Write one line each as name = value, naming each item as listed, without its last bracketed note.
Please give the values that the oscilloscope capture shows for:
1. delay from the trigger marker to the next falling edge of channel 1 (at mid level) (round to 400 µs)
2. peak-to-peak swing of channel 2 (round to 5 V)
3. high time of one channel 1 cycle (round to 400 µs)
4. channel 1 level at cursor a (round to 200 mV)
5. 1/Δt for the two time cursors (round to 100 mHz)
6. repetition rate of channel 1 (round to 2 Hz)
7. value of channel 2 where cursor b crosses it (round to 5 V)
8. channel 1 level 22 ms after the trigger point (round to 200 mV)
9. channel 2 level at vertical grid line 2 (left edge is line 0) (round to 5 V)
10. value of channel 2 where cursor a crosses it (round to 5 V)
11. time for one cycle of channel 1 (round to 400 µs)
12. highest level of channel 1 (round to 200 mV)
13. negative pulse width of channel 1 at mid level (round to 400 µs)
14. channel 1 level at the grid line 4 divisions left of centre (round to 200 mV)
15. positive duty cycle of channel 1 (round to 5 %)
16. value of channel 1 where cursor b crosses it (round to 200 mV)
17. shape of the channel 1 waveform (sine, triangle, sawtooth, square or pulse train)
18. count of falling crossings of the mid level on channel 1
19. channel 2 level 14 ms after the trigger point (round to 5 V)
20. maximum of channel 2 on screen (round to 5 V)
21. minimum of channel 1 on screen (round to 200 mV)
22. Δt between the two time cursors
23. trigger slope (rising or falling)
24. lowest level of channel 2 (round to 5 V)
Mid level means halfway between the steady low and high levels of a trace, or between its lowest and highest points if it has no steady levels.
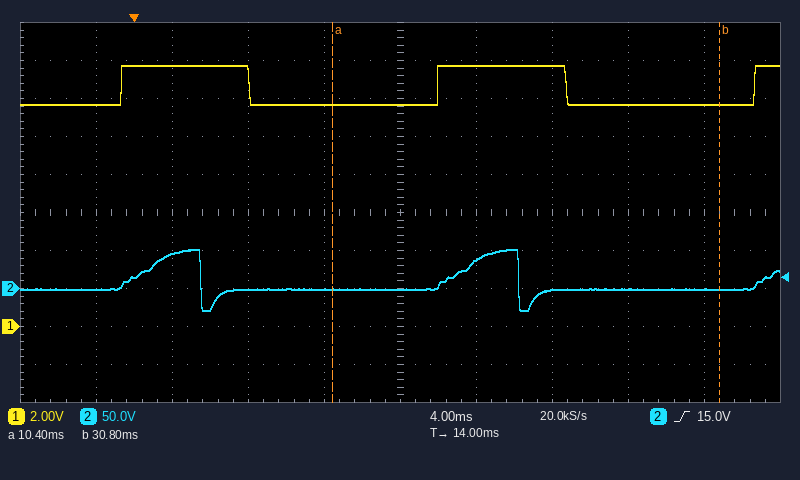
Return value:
delay from the trigger marker to the next falling edge of channel 1 (at mid level) = 6.0 ms
peak-to-peak swing of channel 2 = 80 V
high time of one channel 1 cycle = 6.8 ms
channel 1 level at cursor a = 11.6 V
1/Δt for the two time cursors = 49.0 Hz
repetition rate of channel 1 = 60 Hz
value of channel 2 where cursor b crosses it = 0 V
channel 1 level 22 ms after the trigger point = 13.8 V
channel 2 level at vertical grid line 2 (left edge is line 0) = 45 V
value of channel 2 where cursor a crosses it = 0 V
time for one cycle of channel 1 = 16.8 ms
highest level of channel 1 = 13.8 V
negative pulse width of channel 1 at mid level = 10.0 ms
channel 1 level at the grid line 4 divisions left of centre = 11.6 V
positive duty cycle of channel 1 = 40 %
value of channel 1 where cursor b crosses it = 11.6 V
shape of the channel 1 waveform = pulse train
count of falling crossings of the mid level on channel 1 = 2
channel 2 level 14 ms after the trigger point = 0 V
maximum of channel 2 on screen = 50 V
minimum of channel 1 on screen = 11.6 V
Δt between the two time cursors = 20.4 ms
trigger slope = rising
lowest level of channel 2 = -30 V
